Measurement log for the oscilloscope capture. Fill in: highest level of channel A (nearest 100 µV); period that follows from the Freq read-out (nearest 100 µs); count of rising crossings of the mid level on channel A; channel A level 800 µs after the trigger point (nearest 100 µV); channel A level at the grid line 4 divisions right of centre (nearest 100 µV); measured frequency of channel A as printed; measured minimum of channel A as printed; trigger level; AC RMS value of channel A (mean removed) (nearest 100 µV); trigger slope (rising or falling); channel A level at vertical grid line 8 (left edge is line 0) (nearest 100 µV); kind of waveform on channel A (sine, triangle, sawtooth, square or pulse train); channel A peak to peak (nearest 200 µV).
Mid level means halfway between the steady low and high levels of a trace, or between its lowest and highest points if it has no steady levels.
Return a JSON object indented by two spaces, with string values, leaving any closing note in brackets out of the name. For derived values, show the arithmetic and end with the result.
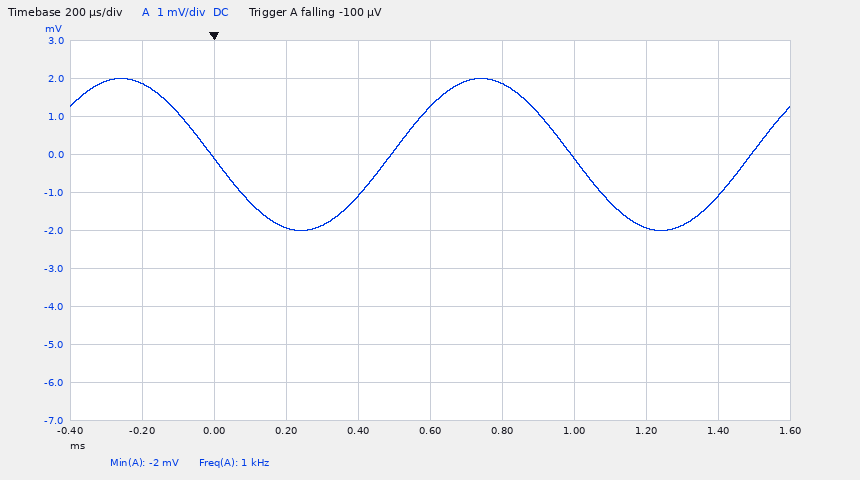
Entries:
{
  "highest level of channel A": "2.0 mV",
  "period that follows from the Freq read-out": "1 / 1 kHz ≈ 1.0 ms",
  "count of rising crossings of the mid level on channel A": "2",
  "channel A level 800 µs after the trigger point": "1.9 mV",
  "channel A level at the grid line 4 divisions right of centre": "-1.1 mV",
  "measured frequency of channel A as printed": "1 kHz",
  "measured minimum of channel A as printed": "-2 mV",
  "trigger level": "-100 µV",
  "AC RMS value of channel A (mean removed)": "4.0 mV / (2√2) ≈ 1.4 mV",
  "trigger slope": "falling",
  "channel A level at vertical grid line 8 (left edge is line 0)": "-1.9 mV",
  "kind of waveform on channel A": "sine",
  "channel A peak to peak": "4.0 mV"
}
